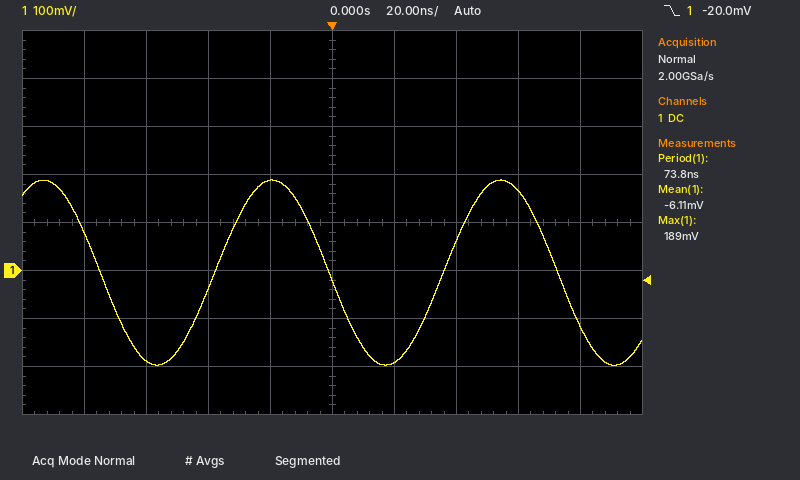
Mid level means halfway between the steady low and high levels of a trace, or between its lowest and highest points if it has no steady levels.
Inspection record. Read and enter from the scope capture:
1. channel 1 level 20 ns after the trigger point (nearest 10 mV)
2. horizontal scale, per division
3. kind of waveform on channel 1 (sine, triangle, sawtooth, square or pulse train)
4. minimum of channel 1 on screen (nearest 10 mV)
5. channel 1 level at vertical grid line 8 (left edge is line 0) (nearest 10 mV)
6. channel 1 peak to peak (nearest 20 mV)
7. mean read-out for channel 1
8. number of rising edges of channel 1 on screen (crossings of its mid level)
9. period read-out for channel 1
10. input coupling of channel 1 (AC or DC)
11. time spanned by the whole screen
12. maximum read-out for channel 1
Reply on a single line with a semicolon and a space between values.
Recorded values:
-190 mV; 20 ns; sine; -200 mV; 170 mV; 380 mV; -6.11 mV; 2; 73.8 ns; DC; 200 ns; 189 mV
